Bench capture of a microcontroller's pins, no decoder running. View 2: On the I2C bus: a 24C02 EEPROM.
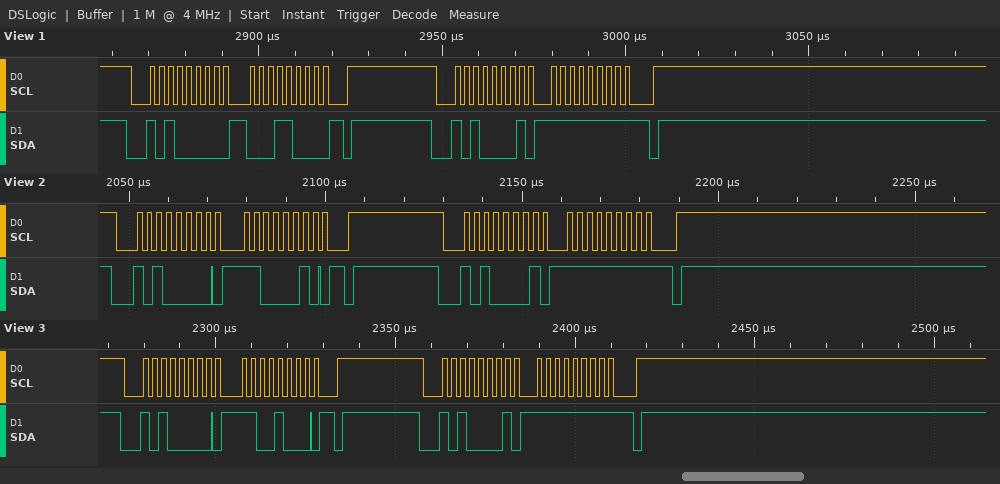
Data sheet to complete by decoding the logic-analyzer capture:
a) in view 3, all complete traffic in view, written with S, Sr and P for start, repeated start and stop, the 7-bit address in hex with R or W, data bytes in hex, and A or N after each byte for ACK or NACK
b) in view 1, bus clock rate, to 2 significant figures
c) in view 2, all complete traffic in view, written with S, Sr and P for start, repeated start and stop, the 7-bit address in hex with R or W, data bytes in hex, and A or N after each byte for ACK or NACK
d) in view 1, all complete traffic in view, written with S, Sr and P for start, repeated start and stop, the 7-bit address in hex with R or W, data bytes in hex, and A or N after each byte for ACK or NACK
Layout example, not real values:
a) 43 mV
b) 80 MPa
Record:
a) S 50W A C8 A P S 50R A FF N P
b) 400 kHz
c) S 50W A C2 A P S 50R A FF N P
d) S 50W A 18 A P S 50R A FF N P
